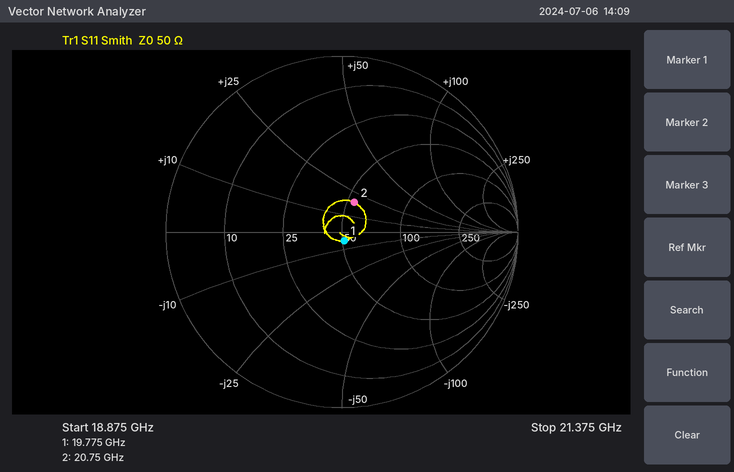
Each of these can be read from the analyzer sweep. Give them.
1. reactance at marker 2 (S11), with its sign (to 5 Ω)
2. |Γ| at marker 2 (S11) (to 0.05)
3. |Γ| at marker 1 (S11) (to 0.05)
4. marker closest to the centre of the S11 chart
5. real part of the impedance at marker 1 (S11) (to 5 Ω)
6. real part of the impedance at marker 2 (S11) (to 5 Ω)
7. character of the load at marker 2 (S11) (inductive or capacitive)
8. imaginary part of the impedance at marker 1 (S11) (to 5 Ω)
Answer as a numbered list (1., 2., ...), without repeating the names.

1. +20 Ω
2. 0.20
3. 0.05
4. marker 1
5. 50 Ω
6. 55 Ω
7. inductive
8. -5 Ω
